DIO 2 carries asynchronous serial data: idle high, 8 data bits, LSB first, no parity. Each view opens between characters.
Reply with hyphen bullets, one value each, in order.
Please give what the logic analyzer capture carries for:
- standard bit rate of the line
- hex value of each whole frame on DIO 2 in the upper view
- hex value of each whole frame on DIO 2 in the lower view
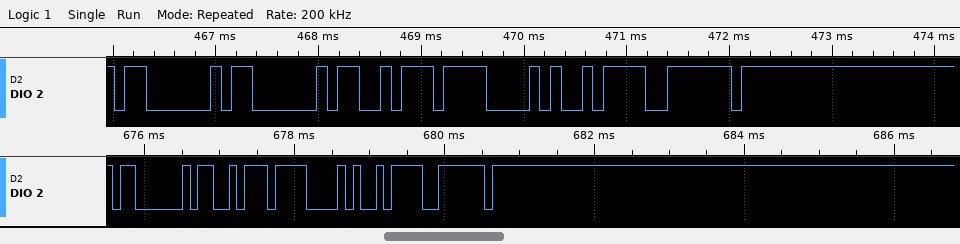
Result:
- 9600 baud
- 03, 03, D3, 0F, E9, 7E
- 03, D3, 0F, E9, 7E
